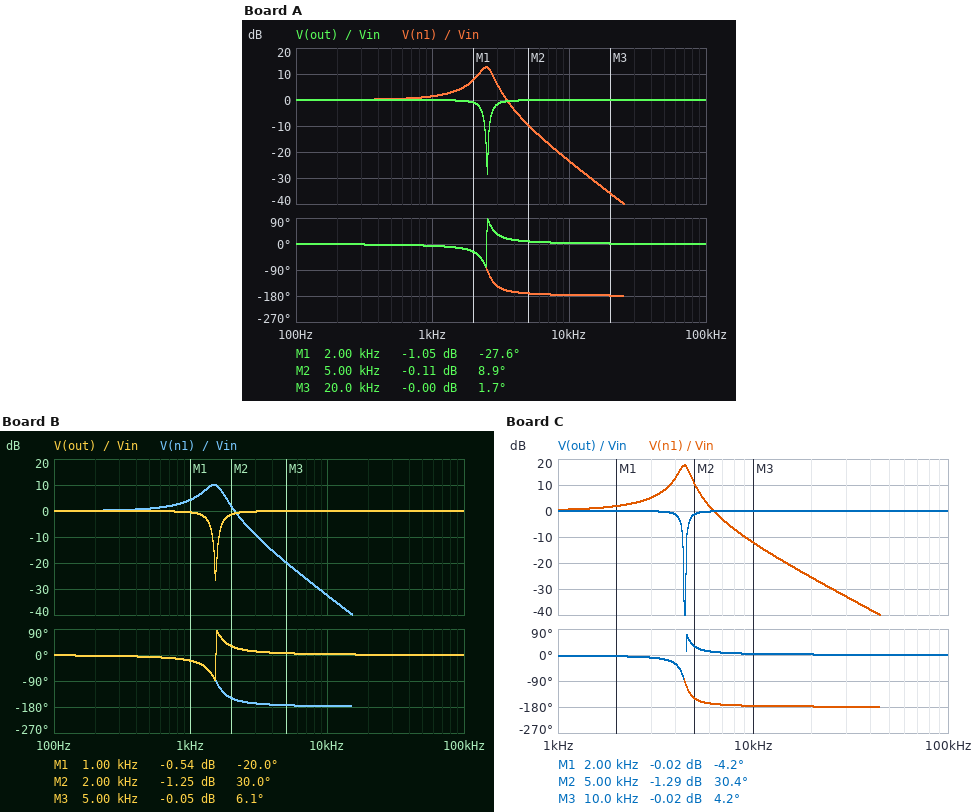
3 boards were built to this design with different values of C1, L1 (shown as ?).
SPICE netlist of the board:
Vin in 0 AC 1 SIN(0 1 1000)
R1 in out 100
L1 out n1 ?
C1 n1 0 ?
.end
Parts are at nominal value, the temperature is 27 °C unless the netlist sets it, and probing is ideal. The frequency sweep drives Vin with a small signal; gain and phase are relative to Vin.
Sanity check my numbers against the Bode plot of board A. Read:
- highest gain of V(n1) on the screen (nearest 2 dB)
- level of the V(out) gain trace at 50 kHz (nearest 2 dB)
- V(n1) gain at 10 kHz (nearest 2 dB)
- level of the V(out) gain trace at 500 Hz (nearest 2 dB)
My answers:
12 dB
0 dB
-24 dB
0 dB
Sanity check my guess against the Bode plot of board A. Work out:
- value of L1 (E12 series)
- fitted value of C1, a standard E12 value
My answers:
27 mH
150 nF
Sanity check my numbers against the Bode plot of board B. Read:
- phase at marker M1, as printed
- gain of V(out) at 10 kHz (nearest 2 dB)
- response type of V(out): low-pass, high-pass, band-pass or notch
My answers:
-20.0 deg
0 dB
notch
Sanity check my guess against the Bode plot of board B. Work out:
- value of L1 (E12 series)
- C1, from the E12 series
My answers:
33 mH
330 nF
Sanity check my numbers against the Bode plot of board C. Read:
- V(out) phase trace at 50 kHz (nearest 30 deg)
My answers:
0 deg
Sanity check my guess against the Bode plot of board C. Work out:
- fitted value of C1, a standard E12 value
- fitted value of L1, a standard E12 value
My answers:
47 nF
27 mH
